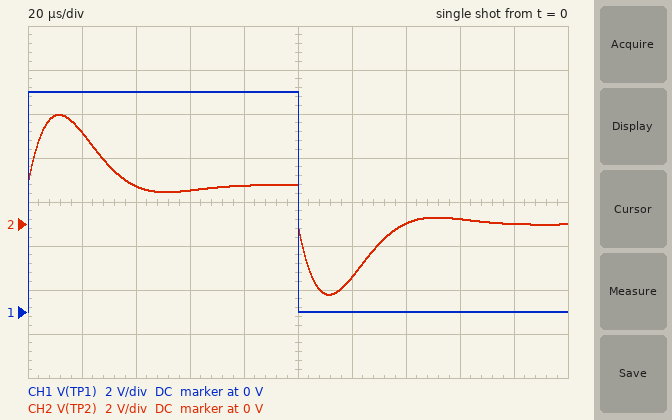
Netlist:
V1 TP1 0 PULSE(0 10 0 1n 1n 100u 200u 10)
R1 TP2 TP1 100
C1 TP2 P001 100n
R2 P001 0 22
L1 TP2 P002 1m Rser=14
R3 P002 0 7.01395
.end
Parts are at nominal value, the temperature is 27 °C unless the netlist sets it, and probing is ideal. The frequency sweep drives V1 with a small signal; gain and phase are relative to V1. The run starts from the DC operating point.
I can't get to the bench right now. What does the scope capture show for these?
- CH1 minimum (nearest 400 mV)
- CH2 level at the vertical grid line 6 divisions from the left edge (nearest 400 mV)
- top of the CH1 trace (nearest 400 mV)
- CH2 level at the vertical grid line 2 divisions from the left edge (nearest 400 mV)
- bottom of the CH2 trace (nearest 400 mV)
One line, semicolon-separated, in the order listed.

0 V; -2.4 V; 10.0 V; 1.6 V; -3.2 V
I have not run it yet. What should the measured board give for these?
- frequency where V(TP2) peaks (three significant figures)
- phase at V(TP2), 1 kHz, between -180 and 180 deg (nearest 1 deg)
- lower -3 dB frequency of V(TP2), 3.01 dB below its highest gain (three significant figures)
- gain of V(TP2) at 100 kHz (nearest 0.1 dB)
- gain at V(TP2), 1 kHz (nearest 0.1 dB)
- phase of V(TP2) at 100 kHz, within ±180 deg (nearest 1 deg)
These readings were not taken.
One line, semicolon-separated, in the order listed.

15.9 kHz; 13 deg; 8.63 kHz; -13.0 dB; -14.8 dB; -27 deg
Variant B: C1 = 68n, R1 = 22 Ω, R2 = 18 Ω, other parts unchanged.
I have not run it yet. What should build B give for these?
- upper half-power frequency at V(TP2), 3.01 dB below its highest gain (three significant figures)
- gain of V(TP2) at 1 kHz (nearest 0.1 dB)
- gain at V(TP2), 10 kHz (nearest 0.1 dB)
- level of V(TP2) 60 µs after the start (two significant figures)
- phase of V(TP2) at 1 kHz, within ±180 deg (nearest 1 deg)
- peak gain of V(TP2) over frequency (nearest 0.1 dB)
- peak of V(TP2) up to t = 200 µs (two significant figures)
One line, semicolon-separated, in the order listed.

89.8 kHz; -5.9 dB; -1.1 dB; 5.3 V; 8 deg; -0.5 dB; 8.7 V
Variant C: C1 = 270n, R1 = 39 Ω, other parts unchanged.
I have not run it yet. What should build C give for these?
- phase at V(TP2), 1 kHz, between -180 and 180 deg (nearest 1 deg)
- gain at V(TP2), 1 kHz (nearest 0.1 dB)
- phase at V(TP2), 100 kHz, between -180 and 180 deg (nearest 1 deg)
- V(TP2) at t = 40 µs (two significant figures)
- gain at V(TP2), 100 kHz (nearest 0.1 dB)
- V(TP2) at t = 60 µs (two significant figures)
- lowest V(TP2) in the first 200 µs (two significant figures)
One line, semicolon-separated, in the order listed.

9 deg; -8.8 dB; -8 deg; 4.9 V; -8.6 dB; 3.9 V; -2.5 V
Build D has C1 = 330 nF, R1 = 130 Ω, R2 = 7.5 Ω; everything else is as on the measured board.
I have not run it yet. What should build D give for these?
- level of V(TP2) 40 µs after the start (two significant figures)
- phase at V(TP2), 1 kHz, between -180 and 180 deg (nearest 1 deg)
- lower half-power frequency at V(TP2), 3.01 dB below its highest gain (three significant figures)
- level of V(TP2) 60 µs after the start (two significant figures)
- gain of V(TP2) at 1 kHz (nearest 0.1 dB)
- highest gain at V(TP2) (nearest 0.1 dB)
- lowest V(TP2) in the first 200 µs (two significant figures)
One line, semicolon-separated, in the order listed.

2.7 V; 12 deg; 5.65 kHz; 1.6 V; -16.7 dB; -6.5 dB; -1.7 V
